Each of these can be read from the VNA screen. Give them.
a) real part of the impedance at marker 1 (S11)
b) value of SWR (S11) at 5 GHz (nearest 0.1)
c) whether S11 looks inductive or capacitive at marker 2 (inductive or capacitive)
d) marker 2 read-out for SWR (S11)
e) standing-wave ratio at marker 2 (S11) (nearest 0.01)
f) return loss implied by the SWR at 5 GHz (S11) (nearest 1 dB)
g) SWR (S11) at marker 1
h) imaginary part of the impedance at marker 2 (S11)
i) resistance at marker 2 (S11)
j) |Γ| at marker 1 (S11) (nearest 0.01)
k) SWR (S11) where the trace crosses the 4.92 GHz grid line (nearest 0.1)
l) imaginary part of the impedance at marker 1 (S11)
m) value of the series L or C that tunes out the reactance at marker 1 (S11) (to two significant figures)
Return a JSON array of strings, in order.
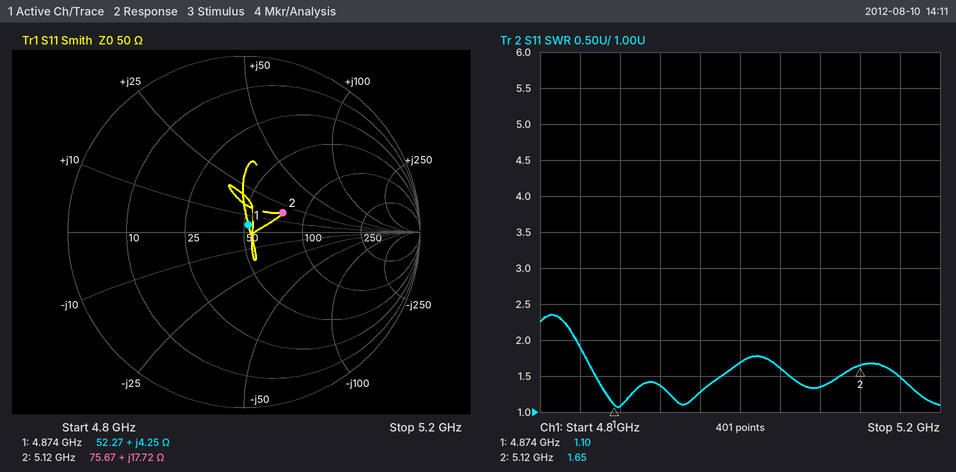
["52.27 Ω", "1.7", "inductive", "1.65", "1.65", "12 dB", "1.10", "+17.72 Ω", "75.67 Ω", "0.05", "1.4", "+4.25 Ω", "7.7 pF"]
